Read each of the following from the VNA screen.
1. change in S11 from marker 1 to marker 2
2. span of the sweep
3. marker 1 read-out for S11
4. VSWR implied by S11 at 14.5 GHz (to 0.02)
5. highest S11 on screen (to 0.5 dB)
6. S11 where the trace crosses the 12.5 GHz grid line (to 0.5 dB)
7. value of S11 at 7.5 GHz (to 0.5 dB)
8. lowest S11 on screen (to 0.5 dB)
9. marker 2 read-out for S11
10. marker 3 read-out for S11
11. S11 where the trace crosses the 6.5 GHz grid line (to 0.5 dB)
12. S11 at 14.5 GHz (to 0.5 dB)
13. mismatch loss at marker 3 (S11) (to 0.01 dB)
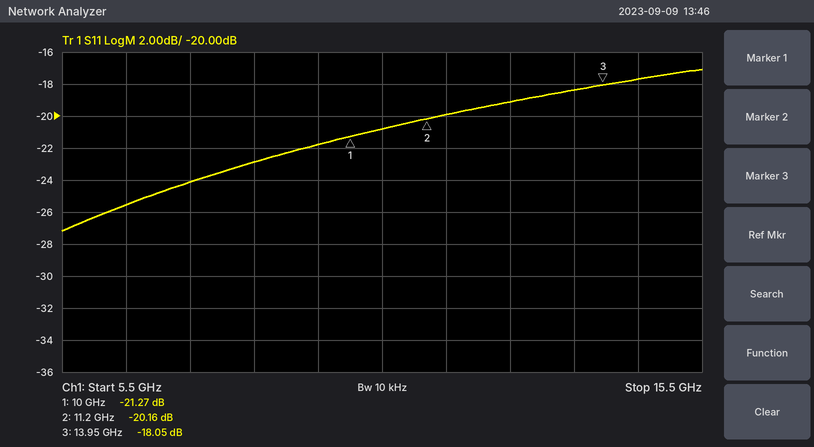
1.11 dB
10 GHz
-21.27 dB
1.30
-17.0 dB
-19.0 dB
-24.0 dB
-27.0 dB
-20.16 dB
-18.05 dB
-25.5 dB
-17.5 dB
0.07 dB
